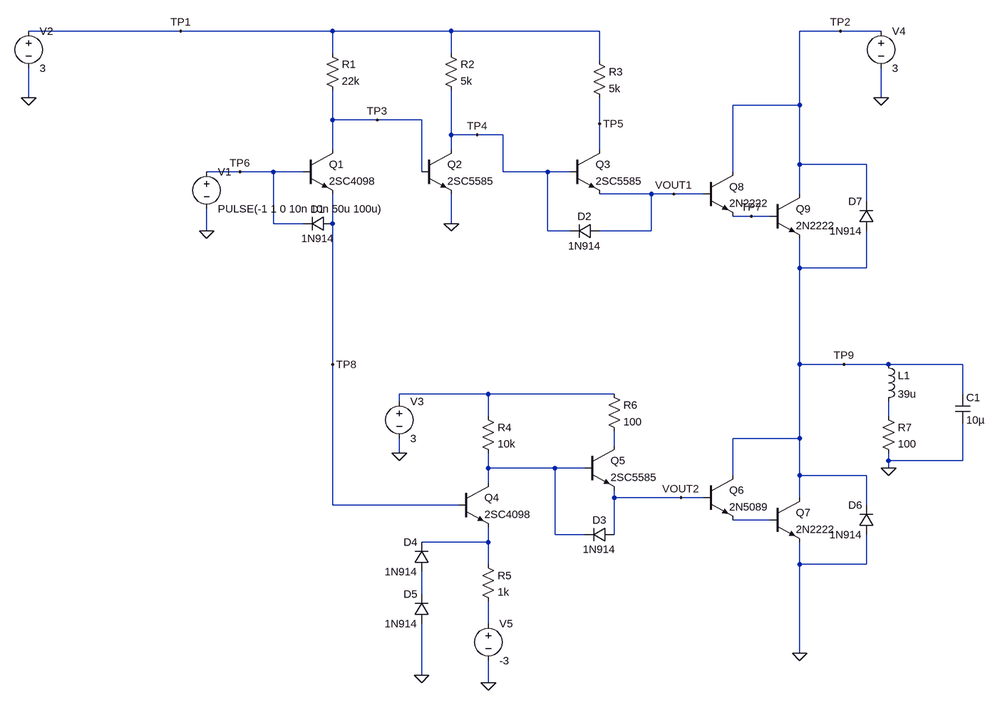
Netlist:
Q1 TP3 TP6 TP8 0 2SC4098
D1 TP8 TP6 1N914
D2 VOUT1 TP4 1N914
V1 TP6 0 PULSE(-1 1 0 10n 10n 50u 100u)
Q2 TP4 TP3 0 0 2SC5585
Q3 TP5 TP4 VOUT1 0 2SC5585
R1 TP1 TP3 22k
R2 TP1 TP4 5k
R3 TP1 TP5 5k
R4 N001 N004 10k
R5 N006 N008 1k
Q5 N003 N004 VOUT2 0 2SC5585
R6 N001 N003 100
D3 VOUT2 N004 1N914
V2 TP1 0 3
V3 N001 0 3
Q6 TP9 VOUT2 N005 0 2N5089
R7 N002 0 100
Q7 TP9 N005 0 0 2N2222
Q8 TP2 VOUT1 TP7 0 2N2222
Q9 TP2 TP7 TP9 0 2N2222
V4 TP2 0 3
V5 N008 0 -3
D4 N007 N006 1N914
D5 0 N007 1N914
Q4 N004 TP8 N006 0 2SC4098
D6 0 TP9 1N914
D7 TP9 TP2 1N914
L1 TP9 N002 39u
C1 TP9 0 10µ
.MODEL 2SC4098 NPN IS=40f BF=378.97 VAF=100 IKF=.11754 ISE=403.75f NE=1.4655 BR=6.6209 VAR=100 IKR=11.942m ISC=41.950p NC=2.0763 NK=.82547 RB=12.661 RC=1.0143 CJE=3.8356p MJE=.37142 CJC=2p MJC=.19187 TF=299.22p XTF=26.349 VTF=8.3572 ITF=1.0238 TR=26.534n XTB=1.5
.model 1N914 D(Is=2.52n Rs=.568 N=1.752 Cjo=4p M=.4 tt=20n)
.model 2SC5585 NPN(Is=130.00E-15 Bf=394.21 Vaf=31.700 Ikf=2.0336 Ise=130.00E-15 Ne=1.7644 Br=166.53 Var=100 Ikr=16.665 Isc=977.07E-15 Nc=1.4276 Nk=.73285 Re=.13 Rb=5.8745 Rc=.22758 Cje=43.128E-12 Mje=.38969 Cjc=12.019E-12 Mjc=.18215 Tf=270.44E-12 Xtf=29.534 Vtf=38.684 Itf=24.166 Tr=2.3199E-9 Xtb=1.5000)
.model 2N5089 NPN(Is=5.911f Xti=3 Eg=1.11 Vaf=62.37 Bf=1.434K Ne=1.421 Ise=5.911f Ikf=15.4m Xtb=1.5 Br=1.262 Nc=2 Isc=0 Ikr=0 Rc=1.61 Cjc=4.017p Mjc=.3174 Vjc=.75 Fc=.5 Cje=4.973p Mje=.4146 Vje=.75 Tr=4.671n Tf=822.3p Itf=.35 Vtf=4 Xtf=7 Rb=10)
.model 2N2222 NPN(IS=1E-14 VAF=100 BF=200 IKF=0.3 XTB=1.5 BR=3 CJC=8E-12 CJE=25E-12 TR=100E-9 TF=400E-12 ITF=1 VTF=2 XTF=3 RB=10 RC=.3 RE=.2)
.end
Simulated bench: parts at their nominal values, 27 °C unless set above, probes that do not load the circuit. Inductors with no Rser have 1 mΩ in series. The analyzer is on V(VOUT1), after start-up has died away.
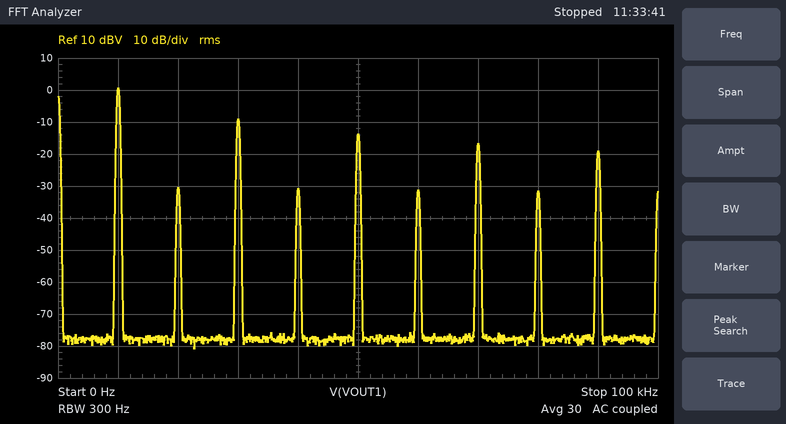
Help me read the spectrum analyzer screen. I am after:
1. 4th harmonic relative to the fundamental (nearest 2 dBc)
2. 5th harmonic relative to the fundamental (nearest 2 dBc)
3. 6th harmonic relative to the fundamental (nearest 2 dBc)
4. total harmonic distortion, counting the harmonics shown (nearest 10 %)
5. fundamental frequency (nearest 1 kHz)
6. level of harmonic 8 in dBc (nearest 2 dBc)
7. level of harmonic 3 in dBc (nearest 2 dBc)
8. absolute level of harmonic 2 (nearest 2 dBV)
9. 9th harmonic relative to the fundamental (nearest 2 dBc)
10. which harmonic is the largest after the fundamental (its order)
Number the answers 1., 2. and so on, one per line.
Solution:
1. -32 dBc
2. -14 dBc
3. -32 dBc
4. 40 %
5. 10 kHz
6. -32 dBc
7. -10 dBc
8. -30 dBV
9. -20 dBc
10. 3
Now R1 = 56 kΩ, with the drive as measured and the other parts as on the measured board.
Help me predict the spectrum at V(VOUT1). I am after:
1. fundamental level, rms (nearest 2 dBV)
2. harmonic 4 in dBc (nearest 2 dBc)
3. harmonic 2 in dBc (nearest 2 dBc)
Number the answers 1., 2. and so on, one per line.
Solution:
1. 0 dBV
2. -24 dBc
3. -24 dBc
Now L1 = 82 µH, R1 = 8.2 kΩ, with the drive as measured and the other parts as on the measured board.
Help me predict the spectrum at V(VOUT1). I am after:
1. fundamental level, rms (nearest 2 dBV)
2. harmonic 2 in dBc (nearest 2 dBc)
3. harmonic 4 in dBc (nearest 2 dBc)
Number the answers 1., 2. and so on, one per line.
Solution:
1. 0 dBV
2. -40 dBc
3. -40 dBc
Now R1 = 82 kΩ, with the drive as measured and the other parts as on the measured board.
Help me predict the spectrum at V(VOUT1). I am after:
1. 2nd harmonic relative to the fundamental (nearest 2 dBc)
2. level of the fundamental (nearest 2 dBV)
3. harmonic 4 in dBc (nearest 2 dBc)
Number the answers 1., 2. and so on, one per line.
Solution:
1. -20 dBc
2. 0 dBV
3. -20 dBc
